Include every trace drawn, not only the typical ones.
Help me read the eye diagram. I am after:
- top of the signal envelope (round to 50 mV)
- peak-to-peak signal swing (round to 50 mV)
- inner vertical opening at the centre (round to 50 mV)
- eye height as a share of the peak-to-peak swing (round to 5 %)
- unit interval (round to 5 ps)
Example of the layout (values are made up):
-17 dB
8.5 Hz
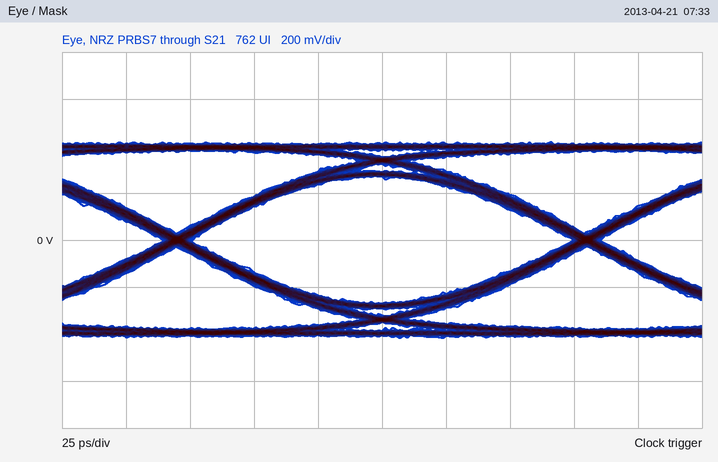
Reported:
400 mV
850 mV
550 mV
65 %
160 ps
